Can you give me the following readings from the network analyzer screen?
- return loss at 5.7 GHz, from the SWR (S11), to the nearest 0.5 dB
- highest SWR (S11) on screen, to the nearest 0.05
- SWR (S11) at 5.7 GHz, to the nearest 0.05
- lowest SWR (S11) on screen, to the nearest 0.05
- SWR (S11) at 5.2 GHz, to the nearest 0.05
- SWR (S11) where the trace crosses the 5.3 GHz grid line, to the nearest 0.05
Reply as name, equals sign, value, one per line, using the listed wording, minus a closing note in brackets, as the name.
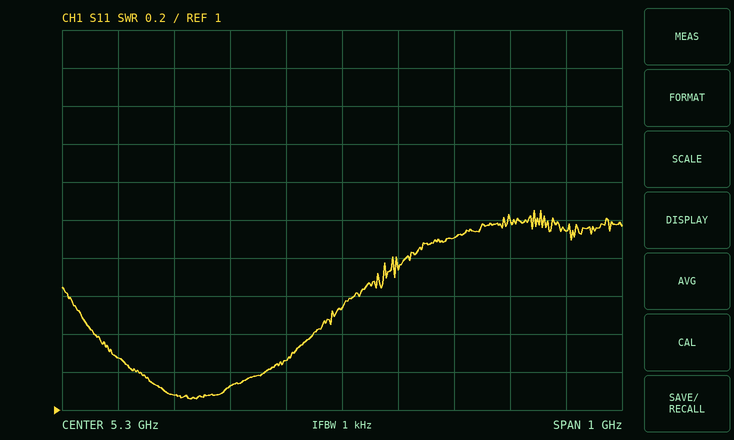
return loss at 5.7 GHz, from the SWR (S11), to the nearest 0.5 dB = 10.0 dB
highest SWR (S11) on screen, to the nearest 0.05 = 2.05
SWR (S11) at 5.7 GHz, to the nearest 0.05 = 1.95
lowest SWR (S11) on screen, to the nearest 0.05 = 1.05
SWR (S11) at 5.2 GHz, to the nearest 0.05 = 1.25
SWR (S11) where the trace crosses the 5.3 GHz grid line, to the nearest 0.05 = 1.55
